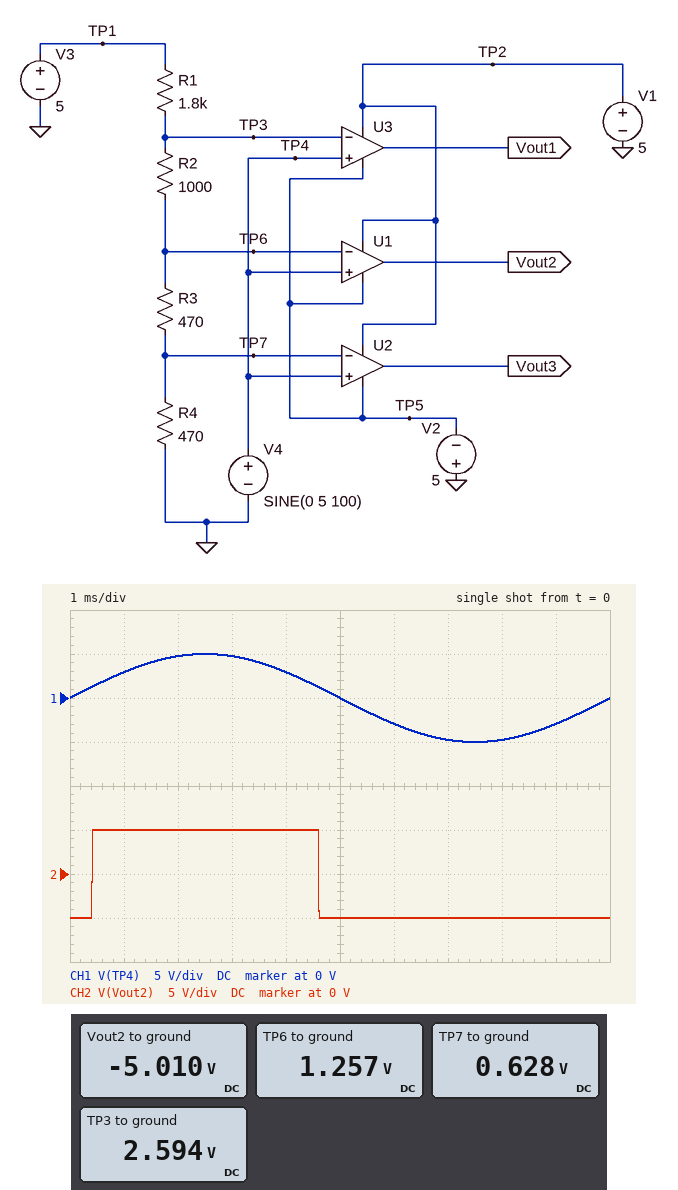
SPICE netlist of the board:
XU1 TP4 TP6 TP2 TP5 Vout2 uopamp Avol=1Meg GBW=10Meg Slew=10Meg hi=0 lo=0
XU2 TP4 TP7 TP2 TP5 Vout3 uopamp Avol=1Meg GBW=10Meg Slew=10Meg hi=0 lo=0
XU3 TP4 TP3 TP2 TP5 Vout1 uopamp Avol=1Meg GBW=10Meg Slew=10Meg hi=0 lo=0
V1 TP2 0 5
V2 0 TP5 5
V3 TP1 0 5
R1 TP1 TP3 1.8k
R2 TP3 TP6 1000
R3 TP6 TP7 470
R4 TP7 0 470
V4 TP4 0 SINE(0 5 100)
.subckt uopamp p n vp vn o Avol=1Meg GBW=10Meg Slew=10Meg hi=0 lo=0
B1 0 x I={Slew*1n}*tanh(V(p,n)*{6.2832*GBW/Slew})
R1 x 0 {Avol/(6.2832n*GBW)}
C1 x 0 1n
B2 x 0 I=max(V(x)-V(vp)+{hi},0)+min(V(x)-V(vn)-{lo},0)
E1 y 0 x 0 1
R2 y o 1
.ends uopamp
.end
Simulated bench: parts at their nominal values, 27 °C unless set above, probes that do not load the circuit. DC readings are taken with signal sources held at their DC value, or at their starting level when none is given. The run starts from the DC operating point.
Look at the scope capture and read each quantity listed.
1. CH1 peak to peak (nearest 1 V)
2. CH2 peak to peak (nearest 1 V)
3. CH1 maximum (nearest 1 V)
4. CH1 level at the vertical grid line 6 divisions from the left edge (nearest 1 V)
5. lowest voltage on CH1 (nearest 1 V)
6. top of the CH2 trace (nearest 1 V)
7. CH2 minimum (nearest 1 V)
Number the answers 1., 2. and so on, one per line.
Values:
1. 10 V
2. 10 V
3. 5 V
4. -3 V
5. -5 V
6. 5 V
7. -5 V
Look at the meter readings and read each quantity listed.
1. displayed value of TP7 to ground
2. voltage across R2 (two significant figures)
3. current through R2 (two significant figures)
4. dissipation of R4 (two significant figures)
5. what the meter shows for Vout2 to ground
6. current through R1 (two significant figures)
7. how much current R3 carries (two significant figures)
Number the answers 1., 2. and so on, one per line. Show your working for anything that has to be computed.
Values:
1. 0.628 V
2. 2.594 V - 1.257 V = 1.3 V
3. (2.594 V - 1.257 V) / 1 kΩ = 1.3 mA
4. (628 mV)^2 / 470 Ω = 840 µW
5. -5.010 V
6. (5 V - 2.594 V) / 1.8 kΩ = 1.3 mA
7. (1.257 V - 628 mV) / 470 Ω = 1.3 mA
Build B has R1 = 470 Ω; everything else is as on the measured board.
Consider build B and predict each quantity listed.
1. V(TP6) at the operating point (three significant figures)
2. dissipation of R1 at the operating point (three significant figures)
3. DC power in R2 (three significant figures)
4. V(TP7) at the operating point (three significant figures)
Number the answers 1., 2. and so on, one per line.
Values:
1. 1.95 V
2. 2.02 mW
3. 4.30 mW
4. 975 mV
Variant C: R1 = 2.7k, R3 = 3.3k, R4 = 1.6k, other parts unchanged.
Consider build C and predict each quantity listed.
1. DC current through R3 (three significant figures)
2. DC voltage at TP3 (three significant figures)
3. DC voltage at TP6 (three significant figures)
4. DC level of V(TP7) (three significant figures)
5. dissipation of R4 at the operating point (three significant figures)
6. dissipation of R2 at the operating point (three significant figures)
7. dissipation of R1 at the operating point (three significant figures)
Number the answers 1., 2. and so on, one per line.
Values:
1. 581 µA
2. 3.43 V
3. 2.85 V
4. 930 mV
5. 541 µW
6. 338 µW
7. 913 µW
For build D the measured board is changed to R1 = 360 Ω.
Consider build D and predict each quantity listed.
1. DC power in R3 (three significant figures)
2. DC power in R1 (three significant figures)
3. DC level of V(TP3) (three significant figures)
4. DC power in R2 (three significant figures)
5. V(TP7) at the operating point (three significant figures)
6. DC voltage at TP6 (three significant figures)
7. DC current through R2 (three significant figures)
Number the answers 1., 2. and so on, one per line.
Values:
1. 2.22 mW
2. 1.70 mW
3. 4.22 V
4. 4.73 mW
5. 1.02 V
6. 2.04 V
7. 2.17 mA
